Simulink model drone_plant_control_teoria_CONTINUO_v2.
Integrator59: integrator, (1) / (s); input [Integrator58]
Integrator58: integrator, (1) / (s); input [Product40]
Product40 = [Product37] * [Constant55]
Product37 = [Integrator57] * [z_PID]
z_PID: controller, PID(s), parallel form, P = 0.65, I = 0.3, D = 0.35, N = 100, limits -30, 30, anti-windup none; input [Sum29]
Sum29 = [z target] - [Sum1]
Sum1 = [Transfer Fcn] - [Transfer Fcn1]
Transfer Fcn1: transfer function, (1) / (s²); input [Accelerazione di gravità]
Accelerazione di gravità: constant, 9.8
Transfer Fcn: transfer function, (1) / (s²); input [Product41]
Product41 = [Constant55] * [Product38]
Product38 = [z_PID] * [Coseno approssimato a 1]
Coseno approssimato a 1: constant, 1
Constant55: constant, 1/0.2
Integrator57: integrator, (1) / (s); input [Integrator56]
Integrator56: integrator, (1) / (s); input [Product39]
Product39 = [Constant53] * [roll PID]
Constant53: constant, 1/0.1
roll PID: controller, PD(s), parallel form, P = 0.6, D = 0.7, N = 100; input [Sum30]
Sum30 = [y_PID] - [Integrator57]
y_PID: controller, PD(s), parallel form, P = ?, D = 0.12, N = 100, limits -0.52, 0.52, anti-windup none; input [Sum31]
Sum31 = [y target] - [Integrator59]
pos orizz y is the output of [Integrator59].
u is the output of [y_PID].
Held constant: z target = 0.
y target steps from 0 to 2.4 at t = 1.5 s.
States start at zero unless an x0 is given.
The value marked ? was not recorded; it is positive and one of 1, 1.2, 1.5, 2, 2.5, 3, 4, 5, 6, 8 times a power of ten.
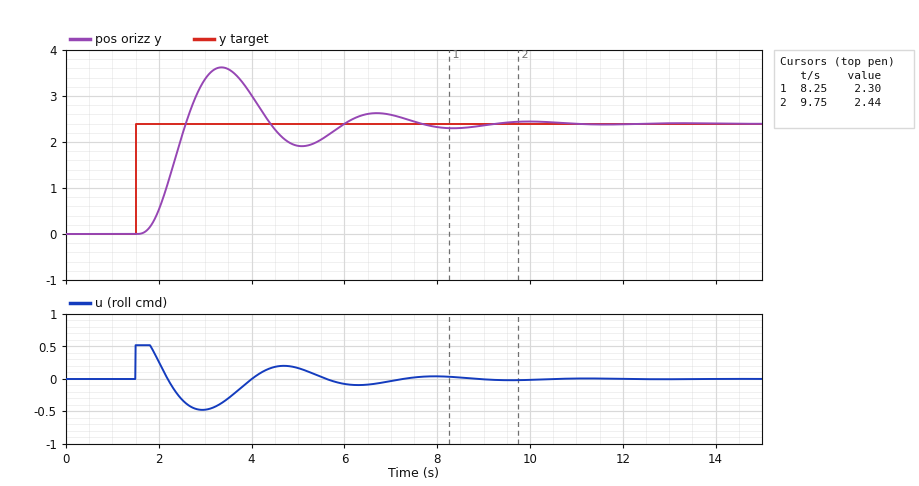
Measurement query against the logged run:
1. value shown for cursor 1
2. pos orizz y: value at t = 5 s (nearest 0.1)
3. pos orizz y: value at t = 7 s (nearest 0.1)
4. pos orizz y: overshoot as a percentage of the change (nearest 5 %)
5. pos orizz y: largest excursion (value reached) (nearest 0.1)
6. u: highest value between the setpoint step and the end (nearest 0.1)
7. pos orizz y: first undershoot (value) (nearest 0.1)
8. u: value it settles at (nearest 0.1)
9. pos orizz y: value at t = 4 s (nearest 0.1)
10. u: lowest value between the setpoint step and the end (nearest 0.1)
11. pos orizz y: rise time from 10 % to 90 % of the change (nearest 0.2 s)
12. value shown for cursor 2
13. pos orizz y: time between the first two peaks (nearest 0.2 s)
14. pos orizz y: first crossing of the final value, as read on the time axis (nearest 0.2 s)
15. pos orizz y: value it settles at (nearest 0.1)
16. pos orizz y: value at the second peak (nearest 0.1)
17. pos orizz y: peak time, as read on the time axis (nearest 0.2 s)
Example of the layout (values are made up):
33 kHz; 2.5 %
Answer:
2.30; 1.9; 2.6; 50 %; 3.6; 0.5; 1.9; 0.0; 3.0; -0.5; 0.6 s; 2.44; 3.4 s; 2.6 s; 2.4; 2.6; 3.4 s
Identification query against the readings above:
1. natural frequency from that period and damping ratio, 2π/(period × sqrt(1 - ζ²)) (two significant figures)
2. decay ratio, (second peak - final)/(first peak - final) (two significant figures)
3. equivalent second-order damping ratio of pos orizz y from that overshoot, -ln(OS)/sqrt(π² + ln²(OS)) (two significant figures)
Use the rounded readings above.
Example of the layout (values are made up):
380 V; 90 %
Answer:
1.9 rad/s; 0.17; 0.22
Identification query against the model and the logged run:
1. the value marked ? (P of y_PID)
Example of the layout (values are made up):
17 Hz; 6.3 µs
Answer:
0.3
